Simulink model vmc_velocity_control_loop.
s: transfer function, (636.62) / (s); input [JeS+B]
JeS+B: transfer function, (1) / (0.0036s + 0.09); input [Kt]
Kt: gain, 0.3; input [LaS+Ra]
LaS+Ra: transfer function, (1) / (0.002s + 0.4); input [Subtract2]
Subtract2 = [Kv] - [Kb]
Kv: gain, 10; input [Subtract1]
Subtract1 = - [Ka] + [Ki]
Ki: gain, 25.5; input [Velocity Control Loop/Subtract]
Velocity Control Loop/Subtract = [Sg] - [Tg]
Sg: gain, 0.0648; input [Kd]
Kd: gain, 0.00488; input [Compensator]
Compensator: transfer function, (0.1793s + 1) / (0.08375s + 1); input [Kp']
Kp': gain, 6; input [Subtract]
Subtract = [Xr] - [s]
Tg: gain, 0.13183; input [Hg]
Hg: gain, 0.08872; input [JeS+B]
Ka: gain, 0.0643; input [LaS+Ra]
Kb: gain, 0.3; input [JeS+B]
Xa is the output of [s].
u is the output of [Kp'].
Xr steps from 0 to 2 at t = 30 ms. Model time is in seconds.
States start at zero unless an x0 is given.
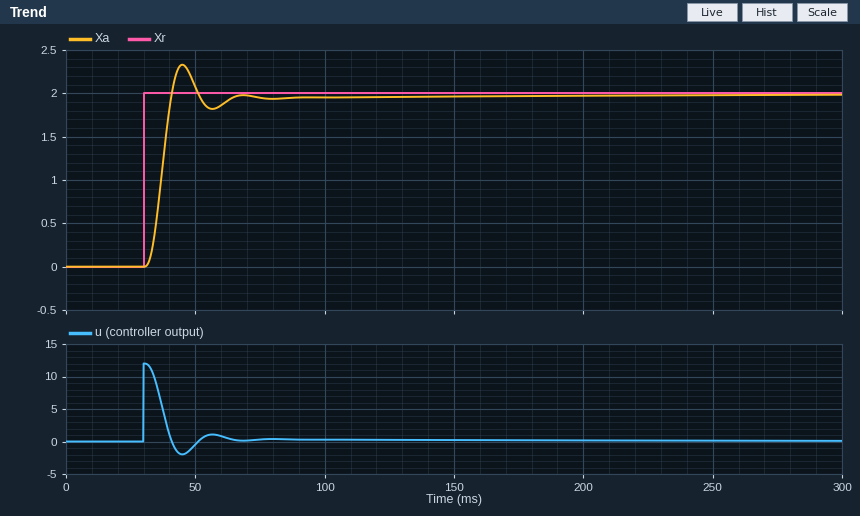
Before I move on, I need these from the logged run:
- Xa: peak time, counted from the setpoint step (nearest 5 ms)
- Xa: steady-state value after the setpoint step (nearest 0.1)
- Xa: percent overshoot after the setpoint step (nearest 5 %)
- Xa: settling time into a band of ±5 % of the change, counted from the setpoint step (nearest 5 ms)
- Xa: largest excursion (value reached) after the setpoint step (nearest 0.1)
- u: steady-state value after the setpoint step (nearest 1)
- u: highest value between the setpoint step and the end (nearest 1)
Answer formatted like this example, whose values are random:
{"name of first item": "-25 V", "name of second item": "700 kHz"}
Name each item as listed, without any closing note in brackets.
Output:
{"Xa: peak time, counted from the setpoint step": "15 ms", "Xa: steady-state value after the setpoint step": "2.0", "Xa: percent overshoot after the setpoint step": "15 %", "Xa: settling time into a band of ±5 % of the change, counted from the setpoint step": "30 ms", "Xa: largest excursion (value reached) after the setpoint step": "2.3", "u: steady-state value after the setpoint step": "0", "u: highest value between the setpoint step and the end": "12"}
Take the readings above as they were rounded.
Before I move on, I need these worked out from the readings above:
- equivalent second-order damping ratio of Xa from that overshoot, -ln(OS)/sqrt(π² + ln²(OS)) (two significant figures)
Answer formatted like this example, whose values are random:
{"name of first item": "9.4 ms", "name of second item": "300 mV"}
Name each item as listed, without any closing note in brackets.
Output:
{"equivalent second-order damping ratio of Xa from that overshoot, -ln(OS)/sqrt(π² + ln²(OS))": "0.52"}
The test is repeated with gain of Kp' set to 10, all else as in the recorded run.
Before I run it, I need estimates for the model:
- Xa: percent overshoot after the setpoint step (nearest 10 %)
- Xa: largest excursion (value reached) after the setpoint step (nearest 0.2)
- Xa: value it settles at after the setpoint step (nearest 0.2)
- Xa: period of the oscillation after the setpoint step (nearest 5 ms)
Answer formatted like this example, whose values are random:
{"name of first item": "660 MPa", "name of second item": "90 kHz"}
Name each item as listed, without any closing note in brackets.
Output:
{"Xa: percent overshoot after the setpoint step": "40 %", "Xa: largest excursion (value reached) after the setpoint step": "2.8", "Xa: value it settles at after the setpoint step": "2.0", "Xa: period of the oscillation after the setpoint step": "20 ms"}
